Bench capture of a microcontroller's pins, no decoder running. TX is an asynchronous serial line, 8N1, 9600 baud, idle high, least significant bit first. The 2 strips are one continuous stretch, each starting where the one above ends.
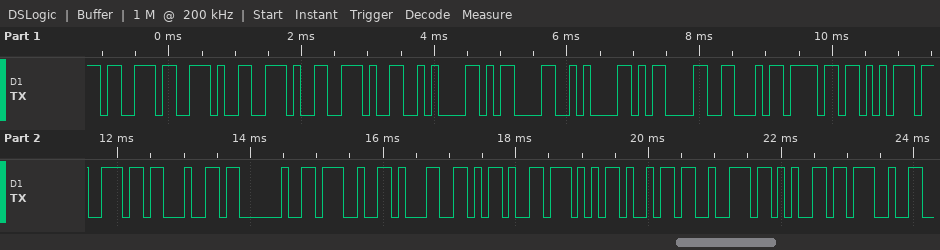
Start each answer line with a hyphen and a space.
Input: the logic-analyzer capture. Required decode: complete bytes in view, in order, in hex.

- 73 2E 2E 2E 0A 0D 0A 0D 46 6F 75 6E 64 20 27 31 2D 57 69 72 65 27
